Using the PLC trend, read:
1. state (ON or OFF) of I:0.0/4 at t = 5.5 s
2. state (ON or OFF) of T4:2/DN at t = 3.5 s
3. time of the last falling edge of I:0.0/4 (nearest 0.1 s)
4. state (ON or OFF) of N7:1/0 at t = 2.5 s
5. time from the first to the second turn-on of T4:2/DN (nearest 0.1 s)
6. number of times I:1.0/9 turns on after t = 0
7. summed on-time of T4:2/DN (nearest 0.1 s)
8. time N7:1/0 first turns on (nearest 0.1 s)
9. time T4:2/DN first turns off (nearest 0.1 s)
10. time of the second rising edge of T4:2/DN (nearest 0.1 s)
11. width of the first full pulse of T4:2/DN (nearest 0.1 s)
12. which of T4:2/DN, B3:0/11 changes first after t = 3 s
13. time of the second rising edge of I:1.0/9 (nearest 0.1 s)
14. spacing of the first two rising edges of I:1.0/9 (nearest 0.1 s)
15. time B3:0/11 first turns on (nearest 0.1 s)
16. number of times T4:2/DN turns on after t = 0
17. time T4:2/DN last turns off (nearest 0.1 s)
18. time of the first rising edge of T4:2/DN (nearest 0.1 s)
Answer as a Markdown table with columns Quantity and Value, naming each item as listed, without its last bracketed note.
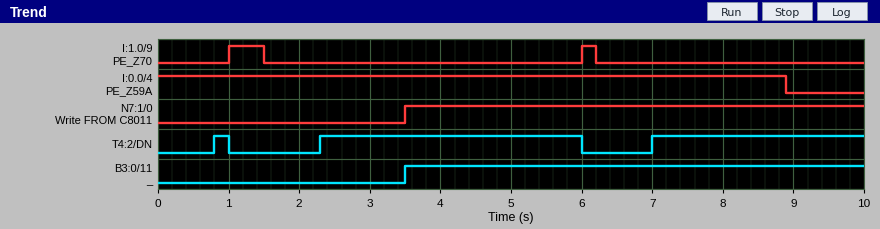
| Quantity | Value |
|---|---|
| state (ON or OFF) of I:0.0/4 at t = 5.5 s | ON |
| state (ON or OFF) of T4:2/DN at t = 3.5 s | ON |
| time of the last falling edge of I:0.0/4 | 8.9 s |
| state (ON or OFF) of N7:1/0 at t = 2.5 s | OFF |
| time from the first to the second turn-on of T4:2/DN | 1.5 s |
| number of times I:1.0/9 turns on after t = 0 | 2 |
| summed on-time of T4:2/DN | 6.9 s |
| time N7:1/0 first turns on | 3.5 s |
| time T4:2/DN first turns off | 1.0 s |
| time of the second rising edge of T4:2/DN | 2.3 s |
| width of the first full pulse of T4:2/DN | 0.2 s |
| which of T4:2/DN, B3:0/11 changes first after t = 3 s | B3:0/11 |
| time of the second rising edge of I:1.0/9 | 6.0 s |
| spacing of the first two rising edges of I:1.0/9 | 5.0 s |
| time B3:0/11 first turns on | 3.5 s |
| number of times T4:2/DN turns on after t = 0 | 3 |
| time T4:2/DN last turns off | 6.0 s |
| time of the first rising edge of T4:2/DN | 0.8 s |
